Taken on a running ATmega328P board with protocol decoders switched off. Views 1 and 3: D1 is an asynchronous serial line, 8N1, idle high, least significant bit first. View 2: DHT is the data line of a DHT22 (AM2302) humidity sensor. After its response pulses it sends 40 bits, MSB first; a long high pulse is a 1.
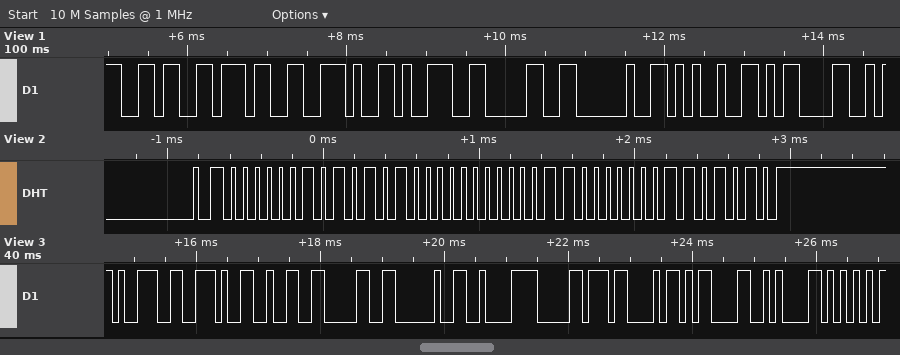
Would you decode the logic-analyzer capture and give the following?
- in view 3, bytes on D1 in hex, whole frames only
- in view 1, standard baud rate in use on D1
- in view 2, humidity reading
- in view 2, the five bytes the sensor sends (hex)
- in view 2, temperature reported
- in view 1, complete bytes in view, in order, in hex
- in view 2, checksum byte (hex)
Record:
39 2E 32 30 20 C2 B0 43 0D 0A 55
9600 baud
68.0 %
02 A8 00 C0 6A
19.2 °C
36 37 2E 39 30 20 25 0D
0x6A
